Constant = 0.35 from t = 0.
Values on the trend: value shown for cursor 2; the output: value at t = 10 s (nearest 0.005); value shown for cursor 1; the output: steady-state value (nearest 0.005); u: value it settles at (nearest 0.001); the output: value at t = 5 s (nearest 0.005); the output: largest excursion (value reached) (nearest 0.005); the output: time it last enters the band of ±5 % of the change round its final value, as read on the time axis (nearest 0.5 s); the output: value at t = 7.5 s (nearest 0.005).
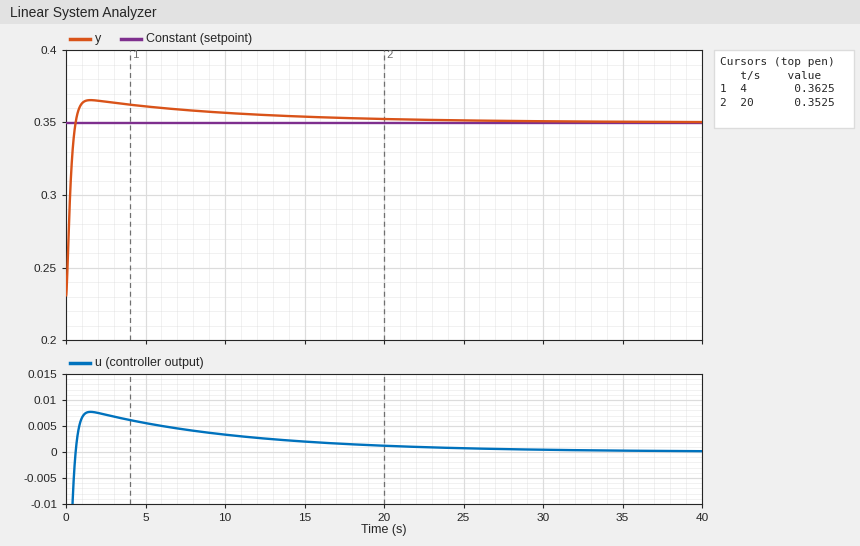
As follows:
0.3525
0.355
0.3625
0.350
0.000
0.360
0.365
11.0 s
0.360
